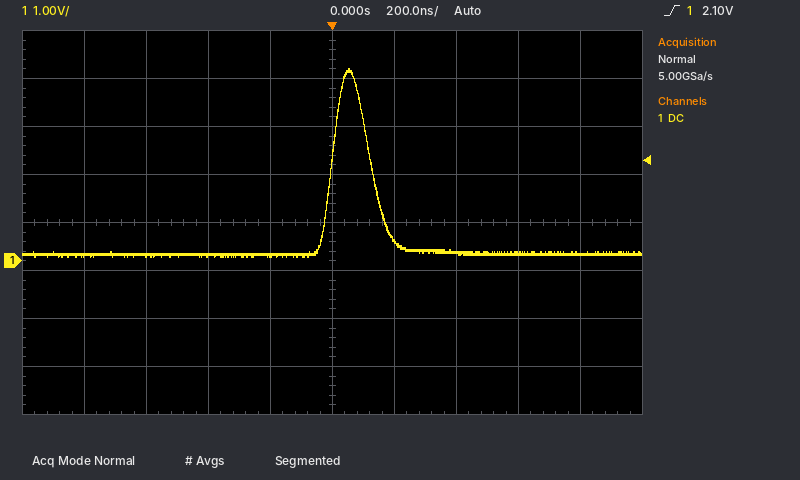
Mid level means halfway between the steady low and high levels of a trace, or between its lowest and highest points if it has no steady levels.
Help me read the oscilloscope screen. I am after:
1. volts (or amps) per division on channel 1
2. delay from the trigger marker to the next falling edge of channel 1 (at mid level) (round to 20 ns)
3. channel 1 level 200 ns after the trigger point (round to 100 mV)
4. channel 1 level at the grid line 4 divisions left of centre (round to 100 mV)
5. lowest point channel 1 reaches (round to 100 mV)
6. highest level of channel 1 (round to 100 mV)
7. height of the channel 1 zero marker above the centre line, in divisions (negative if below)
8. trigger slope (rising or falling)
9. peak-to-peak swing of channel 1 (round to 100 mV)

1 V
120 ns
400 mV
100 mV
100 mV
4.0 V
-0.8 div
rising
3.9 V
